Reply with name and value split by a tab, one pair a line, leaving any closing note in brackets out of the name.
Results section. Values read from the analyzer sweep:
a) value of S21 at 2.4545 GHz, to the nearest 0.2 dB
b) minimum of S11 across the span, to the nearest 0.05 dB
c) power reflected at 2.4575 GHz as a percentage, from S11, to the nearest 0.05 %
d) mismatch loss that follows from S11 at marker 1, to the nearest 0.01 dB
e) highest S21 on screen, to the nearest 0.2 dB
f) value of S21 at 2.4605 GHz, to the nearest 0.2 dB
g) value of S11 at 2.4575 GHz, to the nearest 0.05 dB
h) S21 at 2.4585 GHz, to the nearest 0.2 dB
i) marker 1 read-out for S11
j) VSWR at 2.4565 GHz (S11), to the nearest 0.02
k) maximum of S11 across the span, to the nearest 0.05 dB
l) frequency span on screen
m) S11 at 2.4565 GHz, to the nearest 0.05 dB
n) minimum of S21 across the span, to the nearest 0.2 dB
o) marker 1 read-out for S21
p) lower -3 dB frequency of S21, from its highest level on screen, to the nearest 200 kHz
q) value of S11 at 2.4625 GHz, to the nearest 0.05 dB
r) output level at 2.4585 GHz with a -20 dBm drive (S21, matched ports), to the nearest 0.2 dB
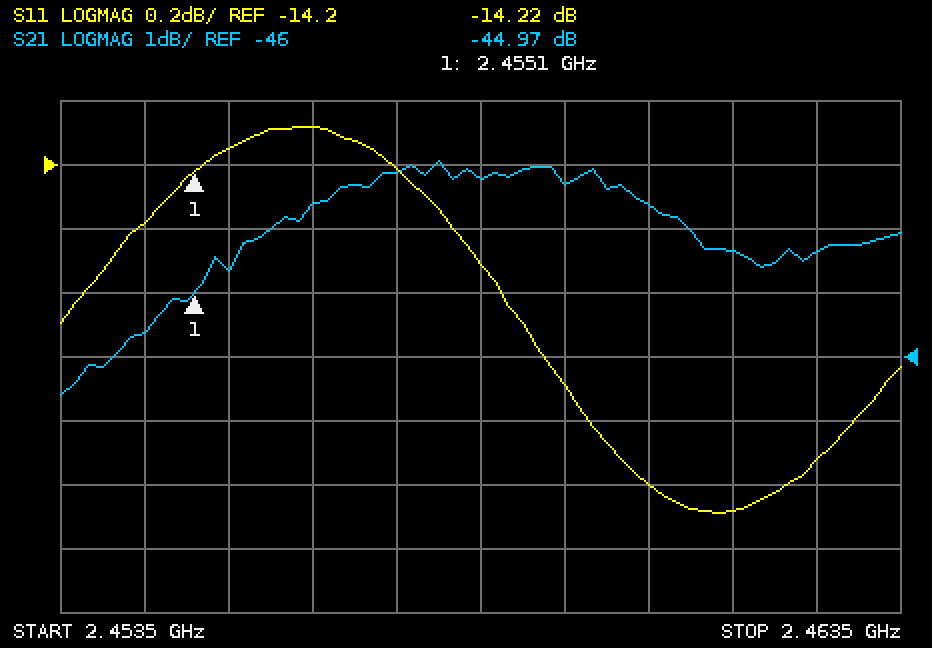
value of S21 at 2.4545 GHz, to the nearest 0.2 dB	-45.6 dB
minimum of S11 across the span, to the nearest 0.05 dB	-15.30 dB
power reflected at 2.4575 GHz as a percentage, from S11, to the nearest 0.05 %	3.80 %
mismatch loss that follows from S11 at marker 1, to the nearest 0.01 dB	0.17 dB
highest S21 on screen, to the nearest 0.2 dB	-43.0 dB
value of S21 at 2.4605 GHz, to the nearest 0.2 dB	-43.6 dB
value of S11 at 2.4575 GHz, to the nearest 0.05 dB	-14.20 dB
S21 at 2.4585 GHz, to the nearest 0.2 dB	-43.2 dB
marker 1 read-out for S11	-14.22 dB
VSWR at 2.4565 GHz (S11), to the nearest 0.02	1.50
maximum of S11 across the span, to the nearest 0.05 dB	-14.10 dB
frequency span on screen	10 MHz
S11 at 2.4565 GHz, to the nearest 0.05 dB	-14.10 dB
minimum of S21 across the span, to the nearest 0.2 dB	-46.6 dB
marker 1 read-out for S21	-44.97 dB
lower -3 dB frequency of S21, from its highest level on screen, to the nearest 200 kHz	2.4542 GHz
value of S11 at 2.4625 GHz, to the nearest 0.05 dB	-15.10 dB
output level at 2.4585 GHz with a -20 dBm drive (S21, matched ports), to the nearest 0.2 dB	-63.2 dBm
